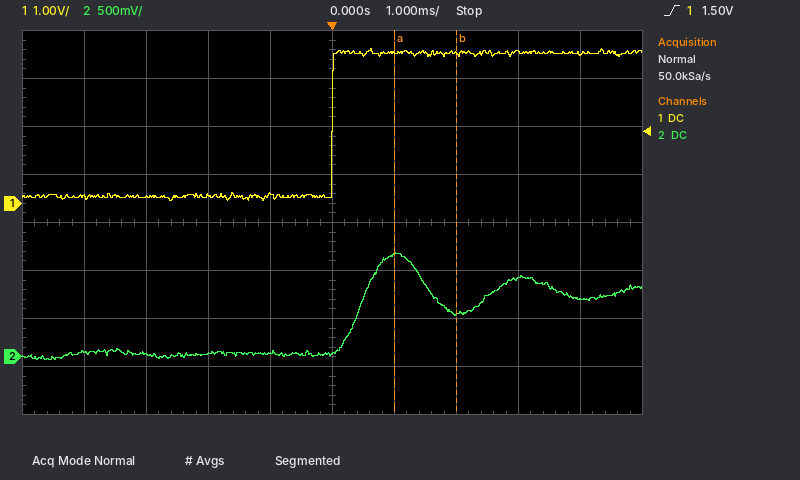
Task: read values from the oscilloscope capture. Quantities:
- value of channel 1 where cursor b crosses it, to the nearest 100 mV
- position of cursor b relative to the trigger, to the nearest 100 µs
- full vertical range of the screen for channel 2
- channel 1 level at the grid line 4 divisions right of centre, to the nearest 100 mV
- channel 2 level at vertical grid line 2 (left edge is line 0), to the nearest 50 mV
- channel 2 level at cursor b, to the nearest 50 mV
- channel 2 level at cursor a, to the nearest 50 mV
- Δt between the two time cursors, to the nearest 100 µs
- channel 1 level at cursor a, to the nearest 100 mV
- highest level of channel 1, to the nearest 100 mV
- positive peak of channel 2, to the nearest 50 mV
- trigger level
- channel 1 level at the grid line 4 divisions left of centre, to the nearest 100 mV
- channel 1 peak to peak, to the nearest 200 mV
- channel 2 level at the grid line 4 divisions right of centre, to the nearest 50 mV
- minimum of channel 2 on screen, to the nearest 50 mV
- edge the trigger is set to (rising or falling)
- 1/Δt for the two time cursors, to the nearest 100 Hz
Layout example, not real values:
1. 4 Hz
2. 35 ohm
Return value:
1. 3.1 V
2. +2.0 ms
3. 4 V
4. 3.1 V
5. 50 mV
6. 450 mV
7. 1.05 V
8. 1.0 ms
9. 3.1 V
10. 3.2 V
11. 1.10 V
12. 1.50 V
13. 100 mV
14. 3.2 V
15. 600 mV
16. -50 mV
17. rising
18. 1.0 kHz
